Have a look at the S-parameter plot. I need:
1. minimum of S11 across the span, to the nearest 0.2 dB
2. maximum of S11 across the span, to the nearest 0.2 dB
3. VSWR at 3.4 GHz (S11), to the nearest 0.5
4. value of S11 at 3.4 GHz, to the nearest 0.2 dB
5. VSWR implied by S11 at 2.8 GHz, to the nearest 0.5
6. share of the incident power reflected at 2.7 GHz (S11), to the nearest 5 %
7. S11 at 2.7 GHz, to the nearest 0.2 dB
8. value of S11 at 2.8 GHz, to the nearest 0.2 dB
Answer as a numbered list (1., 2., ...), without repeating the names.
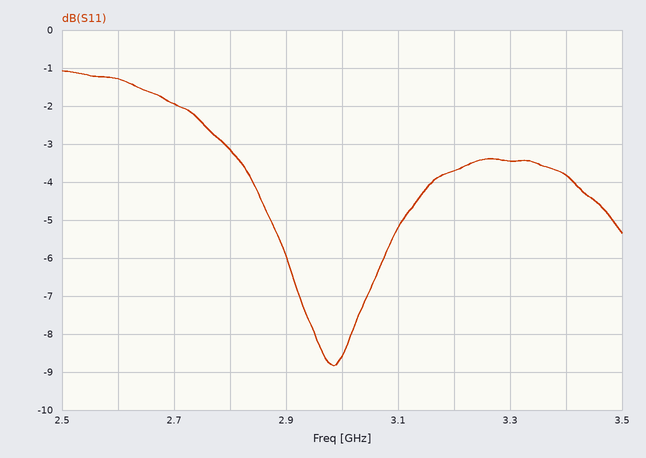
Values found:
1. -8.8 dB
2. -1.0 dB
3. 4.5
4. -3.8 dB
5. 5.5
6. 65 %
7. -2.0 dB
8. -3.2 dB
